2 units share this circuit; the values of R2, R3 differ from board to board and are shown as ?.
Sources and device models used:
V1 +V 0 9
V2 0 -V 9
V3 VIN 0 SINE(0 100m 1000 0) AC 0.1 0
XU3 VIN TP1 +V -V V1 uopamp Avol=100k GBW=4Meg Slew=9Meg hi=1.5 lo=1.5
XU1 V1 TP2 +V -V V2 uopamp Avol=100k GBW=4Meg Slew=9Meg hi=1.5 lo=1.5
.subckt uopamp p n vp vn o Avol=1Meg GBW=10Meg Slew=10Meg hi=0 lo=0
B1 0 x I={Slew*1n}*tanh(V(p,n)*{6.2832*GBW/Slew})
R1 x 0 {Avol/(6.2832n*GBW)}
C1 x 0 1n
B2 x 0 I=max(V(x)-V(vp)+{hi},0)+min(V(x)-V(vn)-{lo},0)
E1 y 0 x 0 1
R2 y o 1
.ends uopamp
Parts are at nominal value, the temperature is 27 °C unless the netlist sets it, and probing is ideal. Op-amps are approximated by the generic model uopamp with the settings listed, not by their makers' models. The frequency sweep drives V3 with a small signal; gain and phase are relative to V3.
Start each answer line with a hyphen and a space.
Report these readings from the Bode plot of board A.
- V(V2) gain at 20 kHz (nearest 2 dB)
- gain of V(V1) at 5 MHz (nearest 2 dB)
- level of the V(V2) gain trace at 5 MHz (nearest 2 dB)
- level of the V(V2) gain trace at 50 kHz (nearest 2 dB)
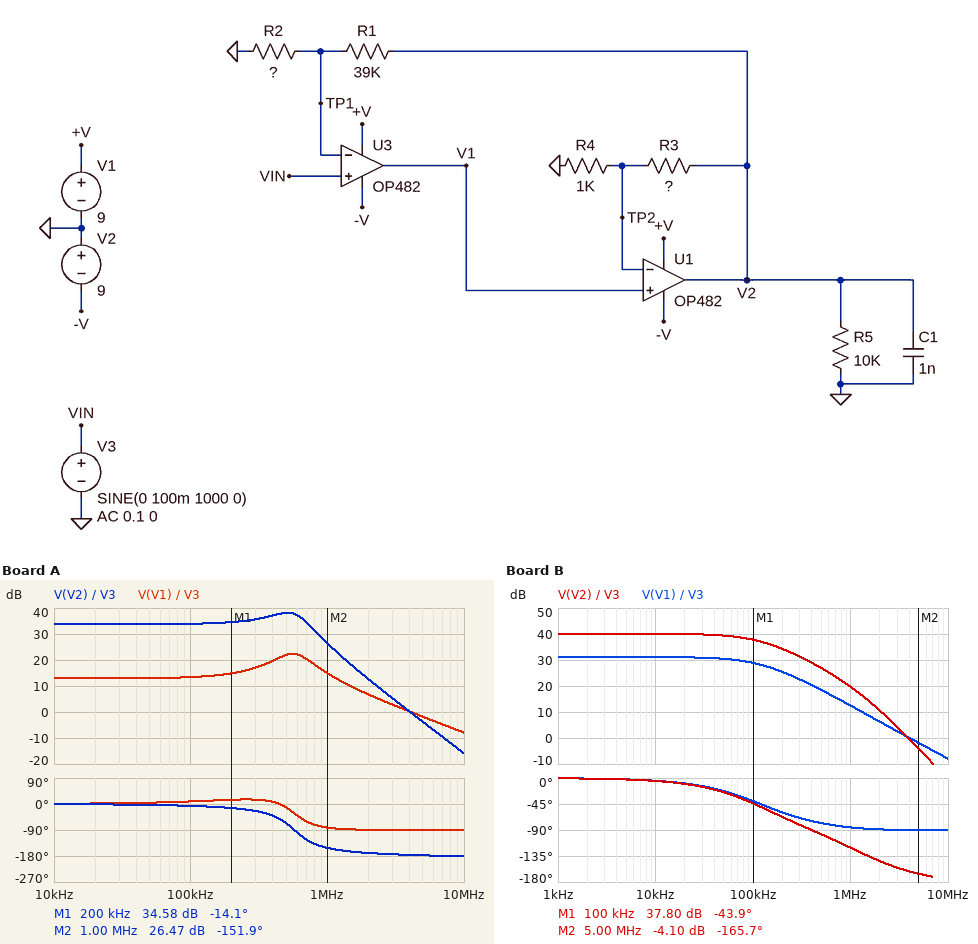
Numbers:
- 34 dB
- -2 dB
- -4 dB
- 34 dB
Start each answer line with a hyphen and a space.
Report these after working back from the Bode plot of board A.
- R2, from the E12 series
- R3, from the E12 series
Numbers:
- 820 Ω
- 10 kΩ
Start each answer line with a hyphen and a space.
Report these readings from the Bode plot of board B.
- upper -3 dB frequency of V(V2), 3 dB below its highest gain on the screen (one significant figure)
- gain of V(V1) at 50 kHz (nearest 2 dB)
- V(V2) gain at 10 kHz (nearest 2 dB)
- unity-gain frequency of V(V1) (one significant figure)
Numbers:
- 100 kHz
- 30 dB
- 40 dB
- 4 MHz
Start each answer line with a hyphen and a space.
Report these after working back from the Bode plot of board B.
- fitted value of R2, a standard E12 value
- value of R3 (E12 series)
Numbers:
- 390 Ω
- 1.8 kΩ
